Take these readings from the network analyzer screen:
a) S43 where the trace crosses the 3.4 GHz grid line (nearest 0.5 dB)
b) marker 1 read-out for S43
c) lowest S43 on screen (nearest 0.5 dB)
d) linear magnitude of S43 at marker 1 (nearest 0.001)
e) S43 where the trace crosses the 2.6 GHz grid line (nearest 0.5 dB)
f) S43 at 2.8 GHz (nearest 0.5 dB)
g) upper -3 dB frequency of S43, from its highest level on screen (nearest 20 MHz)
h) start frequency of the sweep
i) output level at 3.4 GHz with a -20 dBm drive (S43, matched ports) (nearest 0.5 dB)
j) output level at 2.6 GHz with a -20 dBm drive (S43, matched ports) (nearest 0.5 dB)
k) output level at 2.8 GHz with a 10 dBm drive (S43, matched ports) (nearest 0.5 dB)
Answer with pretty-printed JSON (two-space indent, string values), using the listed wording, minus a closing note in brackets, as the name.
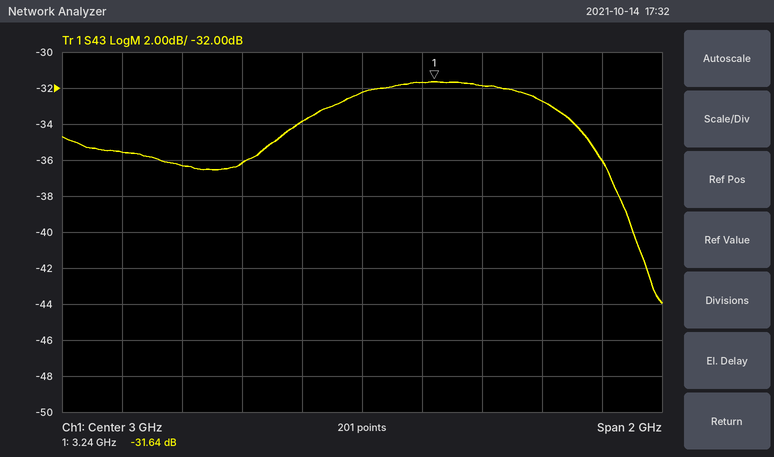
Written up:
{
  "S43 where the trace crosses the 3.4 GHz grid line": "-32.0 dB",
  "marker 1 read-out for S43": "-31.64 dB",
  "lowest S43 on screen": "-44.0 dB",
  "linear magnitude of S43 at marker 1": "0.026",
  "S43 where the trace crosses the 2.6 GHz grid line": "-36.0 dB",
  "S43 at 2.8 GHz": "-34.0 dB",
  "upper -3 dB frequency of S43, from its highest level on screen": "3.74 GHz",
  "start frequency of the sweep": "2 GHz",
  "output level at 3.4 GHz with a -20 dBm drive (S43, matched ports)": "-52.0 dBm",
  "output level at 2.6 GHz with a -20 dBm drive (S43, matched ports)": "-56.0 dBm",
  "output level at 2.8 GHz with a 10 dBm drive (S43, matched ports)": "-24.0 dBm"
}
